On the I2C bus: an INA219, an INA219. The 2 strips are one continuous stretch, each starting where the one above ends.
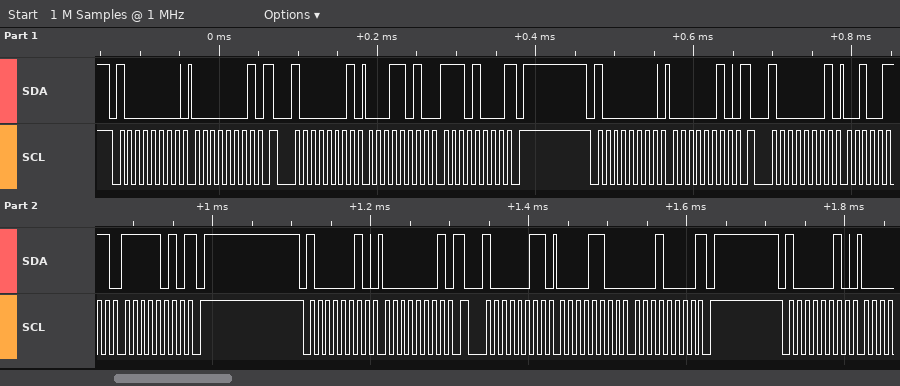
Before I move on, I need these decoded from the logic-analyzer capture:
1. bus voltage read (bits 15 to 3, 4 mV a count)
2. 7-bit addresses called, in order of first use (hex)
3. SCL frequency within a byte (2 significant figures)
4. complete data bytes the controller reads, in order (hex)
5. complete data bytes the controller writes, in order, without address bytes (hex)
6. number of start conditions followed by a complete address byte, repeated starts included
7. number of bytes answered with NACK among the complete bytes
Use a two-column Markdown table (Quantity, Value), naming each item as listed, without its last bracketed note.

| Quantity | Value |
|---|---|
| bus voltage read | 5.116 V |
| 7-bit addresses called, in order of first use | 0x40 0x41 |
| SCL frequency within a byte | 100 kHz |
| complete data bytes the controller reads, in order | 1A E8 27 FA 0C 10 |
| complete data bytes the controller writes, in order, without address bytes | 01 02 01 |
| number of start conditions followed by a complete address byte, repeated starts included | 7 |
| number of bytes answered with NACK among the complete bytes | 3 |
